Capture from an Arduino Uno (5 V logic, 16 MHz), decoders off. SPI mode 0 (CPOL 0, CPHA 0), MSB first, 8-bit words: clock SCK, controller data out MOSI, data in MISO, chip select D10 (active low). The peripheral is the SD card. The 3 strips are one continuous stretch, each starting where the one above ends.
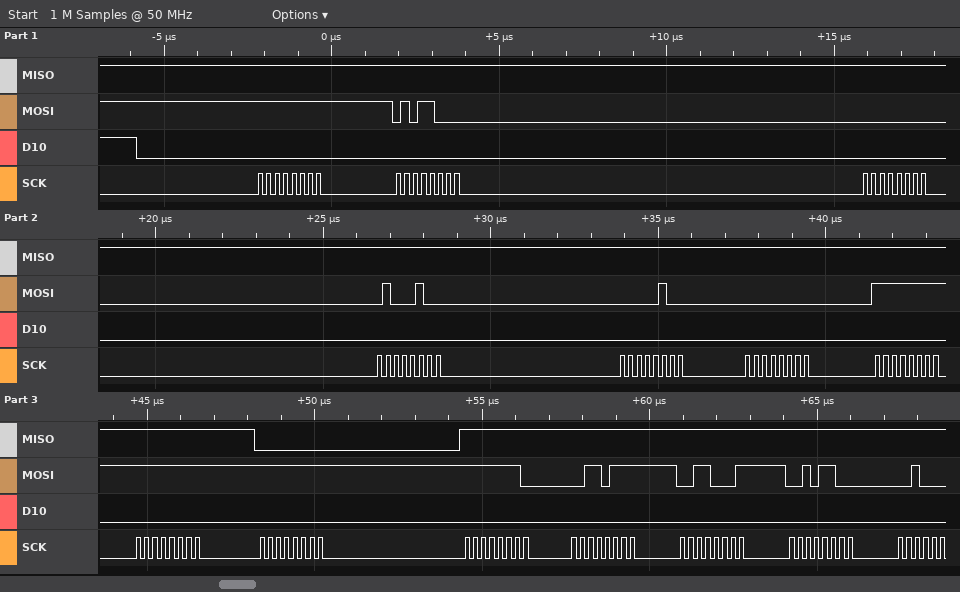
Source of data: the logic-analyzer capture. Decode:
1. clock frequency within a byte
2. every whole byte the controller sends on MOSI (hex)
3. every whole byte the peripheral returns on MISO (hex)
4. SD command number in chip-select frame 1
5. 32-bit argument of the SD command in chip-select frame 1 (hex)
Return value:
4 MHz
0xFF 0x58 0x00 0x44 0x04 0x00 0xFF 0xFF 0xFF 0xFE 0x37 0x31 0x2C
0xFF 0xFF 0xFF 0xFF 0xFF 0xFF 0xFF 0xFF 0x00 0xFF 0xFF 0xFF 0xFF
CMD24
0x00440400
